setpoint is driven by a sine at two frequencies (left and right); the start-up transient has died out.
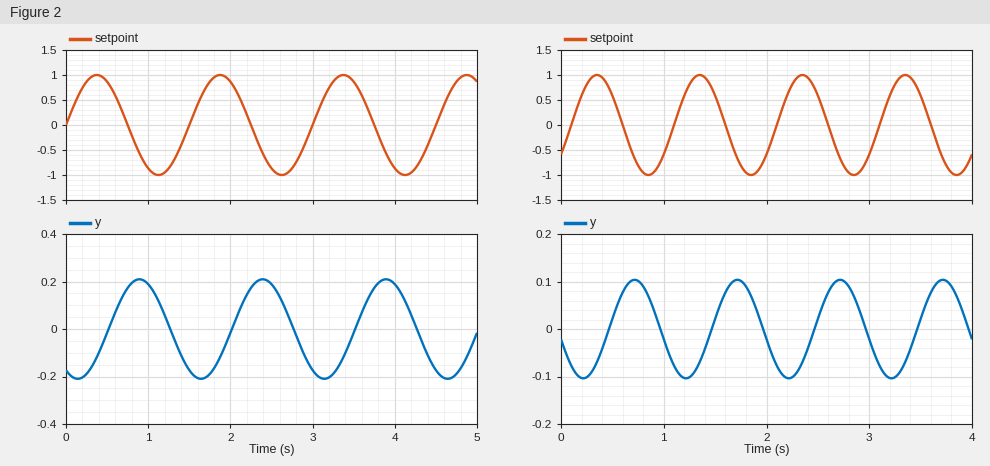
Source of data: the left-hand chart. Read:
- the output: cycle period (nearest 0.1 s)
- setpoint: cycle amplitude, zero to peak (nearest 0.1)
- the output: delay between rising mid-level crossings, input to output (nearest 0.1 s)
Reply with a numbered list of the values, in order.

1. 1.5 s
2. 1.0
3. 0.5 s
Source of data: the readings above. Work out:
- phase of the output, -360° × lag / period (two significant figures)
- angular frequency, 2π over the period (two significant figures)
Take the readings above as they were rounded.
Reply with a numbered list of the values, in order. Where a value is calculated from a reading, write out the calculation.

1. -360 × 0.5 / 1.5 = -120°
2. 2π / 1.5 = 4.2 rad/s
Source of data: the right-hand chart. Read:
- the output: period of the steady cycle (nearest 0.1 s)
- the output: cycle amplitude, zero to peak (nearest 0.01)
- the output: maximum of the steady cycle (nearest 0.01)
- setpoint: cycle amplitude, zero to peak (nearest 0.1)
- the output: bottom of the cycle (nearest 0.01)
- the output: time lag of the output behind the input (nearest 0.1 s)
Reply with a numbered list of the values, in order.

1. 1.0 s
2. 0.10
3. 0.10
4. 1.0
5. -0.10
6. 0.4 s
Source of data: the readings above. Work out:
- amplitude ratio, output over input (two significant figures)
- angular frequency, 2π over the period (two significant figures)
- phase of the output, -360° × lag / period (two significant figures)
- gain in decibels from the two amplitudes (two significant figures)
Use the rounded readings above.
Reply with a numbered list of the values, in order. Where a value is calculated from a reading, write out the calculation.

1. 0.1 / 1 = 0.10
2. 2π / 1 = 6.3 rad/s
3. -360 × 0.4 / 1 = -140°
4. 20 log10(0.1 / 1) = -20 dB
